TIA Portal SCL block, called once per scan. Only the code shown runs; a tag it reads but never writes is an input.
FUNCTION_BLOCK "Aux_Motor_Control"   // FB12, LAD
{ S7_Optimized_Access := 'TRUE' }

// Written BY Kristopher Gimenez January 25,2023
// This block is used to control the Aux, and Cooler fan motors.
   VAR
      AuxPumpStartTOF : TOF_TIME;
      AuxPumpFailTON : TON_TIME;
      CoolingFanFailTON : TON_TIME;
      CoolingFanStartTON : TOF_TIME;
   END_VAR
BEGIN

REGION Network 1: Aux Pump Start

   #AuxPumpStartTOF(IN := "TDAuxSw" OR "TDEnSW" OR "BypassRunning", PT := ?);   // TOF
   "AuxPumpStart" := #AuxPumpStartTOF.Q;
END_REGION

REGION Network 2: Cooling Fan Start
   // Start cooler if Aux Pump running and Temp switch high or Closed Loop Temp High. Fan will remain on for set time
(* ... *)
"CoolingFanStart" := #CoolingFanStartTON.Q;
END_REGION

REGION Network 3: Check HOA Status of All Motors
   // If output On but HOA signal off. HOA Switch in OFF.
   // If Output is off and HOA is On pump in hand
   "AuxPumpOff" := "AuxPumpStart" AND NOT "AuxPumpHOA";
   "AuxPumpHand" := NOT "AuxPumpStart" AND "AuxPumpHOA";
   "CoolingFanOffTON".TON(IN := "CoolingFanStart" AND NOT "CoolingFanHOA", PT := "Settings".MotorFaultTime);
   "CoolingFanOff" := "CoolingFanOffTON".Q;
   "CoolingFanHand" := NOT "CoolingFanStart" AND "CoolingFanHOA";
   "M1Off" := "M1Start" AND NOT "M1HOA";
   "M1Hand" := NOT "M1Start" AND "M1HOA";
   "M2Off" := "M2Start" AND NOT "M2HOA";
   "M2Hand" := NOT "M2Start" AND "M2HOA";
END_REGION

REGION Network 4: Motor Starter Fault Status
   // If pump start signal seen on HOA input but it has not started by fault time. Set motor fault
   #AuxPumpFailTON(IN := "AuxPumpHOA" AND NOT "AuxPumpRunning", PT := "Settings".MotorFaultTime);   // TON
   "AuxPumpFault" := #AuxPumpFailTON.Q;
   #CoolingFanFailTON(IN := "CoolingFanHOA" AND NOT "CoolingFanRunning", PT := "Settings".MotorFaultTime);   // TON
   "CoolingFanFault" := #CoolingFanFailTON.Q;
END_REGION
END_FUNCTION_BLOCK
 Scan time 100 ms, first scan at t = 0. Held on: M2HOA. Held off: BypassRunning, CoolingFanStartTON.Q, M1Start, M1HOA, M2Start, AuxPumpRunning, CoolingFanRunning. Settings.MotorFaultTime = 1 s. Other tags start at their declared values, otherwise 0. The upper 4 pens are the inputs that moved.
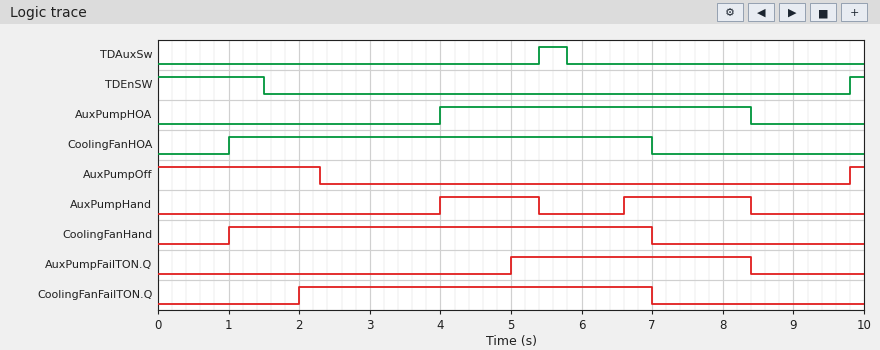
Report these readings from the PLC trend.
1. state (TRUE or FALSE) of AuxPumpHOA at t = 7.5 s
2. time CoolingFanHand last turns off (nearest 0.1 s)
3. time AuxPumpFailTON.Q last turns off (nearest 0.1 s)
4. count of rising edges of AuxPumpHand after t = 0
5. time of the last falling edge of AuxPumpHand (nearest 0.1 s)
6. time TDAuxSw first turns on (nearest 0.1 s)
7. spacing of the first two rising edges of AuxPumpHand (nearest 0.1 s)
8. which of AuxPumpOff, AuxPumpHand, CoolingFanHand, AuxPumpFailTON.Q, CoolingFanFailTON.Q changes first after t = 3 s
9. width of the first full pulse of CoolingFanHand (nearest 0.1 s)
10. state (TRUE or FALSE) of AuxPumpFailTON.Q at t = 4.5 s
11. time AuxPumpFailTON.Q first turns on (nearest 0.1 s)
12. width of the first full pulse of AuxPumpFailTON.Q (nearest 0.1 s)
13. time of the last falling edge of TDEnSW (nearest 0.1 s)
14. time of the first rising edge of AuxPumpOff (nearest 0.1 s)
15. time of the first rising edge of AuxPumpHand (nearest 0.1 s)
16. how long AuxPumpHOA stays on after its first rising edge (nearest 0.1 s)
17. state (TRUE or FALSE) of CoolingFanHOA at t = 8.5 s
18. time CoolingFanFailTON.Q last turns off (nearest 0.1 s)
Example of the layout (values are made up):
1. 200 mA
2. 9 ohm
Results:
1. TRUE
2. 7.0 s
3. 8.4 s
4. 2
5. 8.4 s
6. 5.4 s
7. 2.6 s
8. AuxPumpHand
9. 6.0 s
10. FALSE
11. 5.0 s
12. 3.4 s
13. 1.5 s
14. 9.8 s
15. 4.0 s
16. 4.4 s
17. FALSE
18. 7.0 s
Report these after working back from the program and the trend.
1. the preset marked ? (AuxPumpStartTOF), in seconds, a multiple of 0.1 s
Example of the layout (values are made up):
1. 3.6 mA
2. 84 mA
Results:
1. 0.8 s
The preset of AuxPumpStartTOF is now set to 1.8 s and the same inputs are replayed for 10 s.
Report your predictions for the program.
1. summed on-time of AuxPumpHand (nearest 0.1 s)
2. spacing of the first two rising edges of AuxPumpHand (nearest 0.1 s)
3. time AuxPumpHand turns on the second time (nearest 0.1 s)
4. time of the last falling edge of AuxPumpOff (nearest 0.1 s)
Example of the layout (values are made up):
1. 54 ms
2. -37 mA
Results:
1. 2.2 s
2. 3.6 s
3. 7.6 s
4. 3.3 s
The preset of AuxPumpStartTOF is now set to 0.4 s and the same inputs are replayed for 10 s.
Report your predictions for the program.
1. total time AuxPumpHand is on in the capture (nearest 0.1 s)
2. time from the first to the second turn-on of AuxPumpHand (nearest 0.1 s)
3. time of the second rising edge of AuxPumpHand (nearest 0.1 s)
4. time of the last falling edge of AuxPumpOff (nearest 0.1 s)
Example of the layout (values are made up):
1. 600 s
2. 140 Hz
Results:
1. 3.6 s
2. 2.2 s
3. 6.2 s
4. 1.9 s
